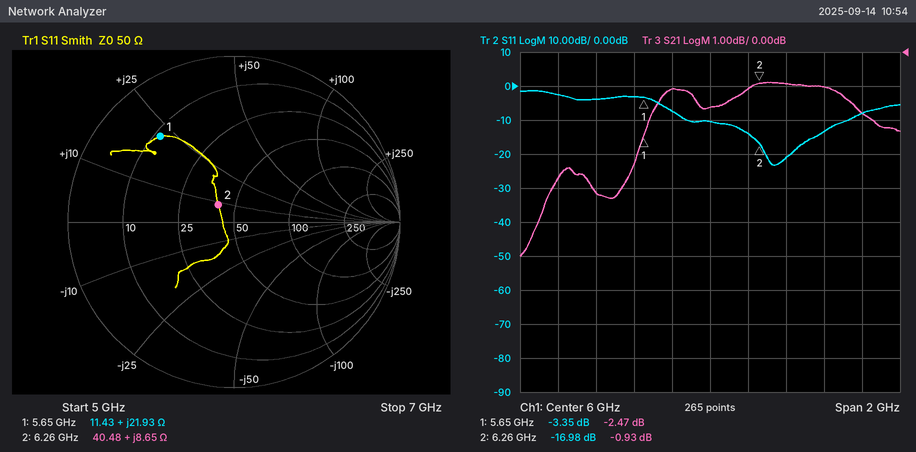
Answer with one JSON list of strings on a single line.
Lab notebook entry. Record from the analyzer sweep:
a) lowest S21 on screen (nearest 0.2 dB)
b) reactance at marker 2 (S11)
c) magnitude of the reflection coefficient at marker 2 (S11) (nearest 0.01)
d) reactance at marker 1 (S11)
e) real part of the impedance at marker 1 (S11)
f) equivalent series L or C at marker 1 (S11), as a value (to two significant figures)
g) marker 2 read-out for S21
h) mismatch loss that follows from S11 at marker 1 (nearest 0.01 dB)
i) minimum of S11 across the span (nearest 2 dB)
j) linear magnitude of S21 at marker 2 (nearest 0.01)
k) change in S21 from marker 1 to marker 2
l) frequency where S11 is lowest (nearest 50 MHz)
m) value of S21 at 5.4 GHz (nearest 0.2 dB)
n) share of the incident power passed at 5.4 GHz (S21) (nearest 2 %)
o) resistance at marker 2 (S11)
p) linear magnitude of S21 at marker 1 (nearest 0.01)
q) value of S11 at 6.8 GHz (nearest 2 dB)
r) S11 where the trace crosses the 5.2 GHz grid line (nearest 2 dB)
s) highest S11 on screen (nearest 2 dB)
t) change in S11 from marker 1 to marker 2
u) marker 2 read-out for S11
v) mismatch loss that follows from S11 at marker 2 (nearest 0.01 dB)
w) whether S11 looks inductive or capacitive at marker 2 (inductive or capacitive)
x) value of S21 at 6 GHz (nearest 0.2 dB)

["-6.0 dB", "+8.65 Ω", "0.14", "+21.93 Ω", "11.43 Ω", "620 pH", "-0.93 dB", "2.70 dB", "-24 dB", "0.90", "1.54 dB", "6.35 GHz", "-4.2 dB", "38 %", "40.48 Ω", "0.75", "-8 dB", "-2 dB", "-2 dB", "-13.63 dB", "-16.98 dB", "0.09 dB", "inductive", "-1.6 dB"]
